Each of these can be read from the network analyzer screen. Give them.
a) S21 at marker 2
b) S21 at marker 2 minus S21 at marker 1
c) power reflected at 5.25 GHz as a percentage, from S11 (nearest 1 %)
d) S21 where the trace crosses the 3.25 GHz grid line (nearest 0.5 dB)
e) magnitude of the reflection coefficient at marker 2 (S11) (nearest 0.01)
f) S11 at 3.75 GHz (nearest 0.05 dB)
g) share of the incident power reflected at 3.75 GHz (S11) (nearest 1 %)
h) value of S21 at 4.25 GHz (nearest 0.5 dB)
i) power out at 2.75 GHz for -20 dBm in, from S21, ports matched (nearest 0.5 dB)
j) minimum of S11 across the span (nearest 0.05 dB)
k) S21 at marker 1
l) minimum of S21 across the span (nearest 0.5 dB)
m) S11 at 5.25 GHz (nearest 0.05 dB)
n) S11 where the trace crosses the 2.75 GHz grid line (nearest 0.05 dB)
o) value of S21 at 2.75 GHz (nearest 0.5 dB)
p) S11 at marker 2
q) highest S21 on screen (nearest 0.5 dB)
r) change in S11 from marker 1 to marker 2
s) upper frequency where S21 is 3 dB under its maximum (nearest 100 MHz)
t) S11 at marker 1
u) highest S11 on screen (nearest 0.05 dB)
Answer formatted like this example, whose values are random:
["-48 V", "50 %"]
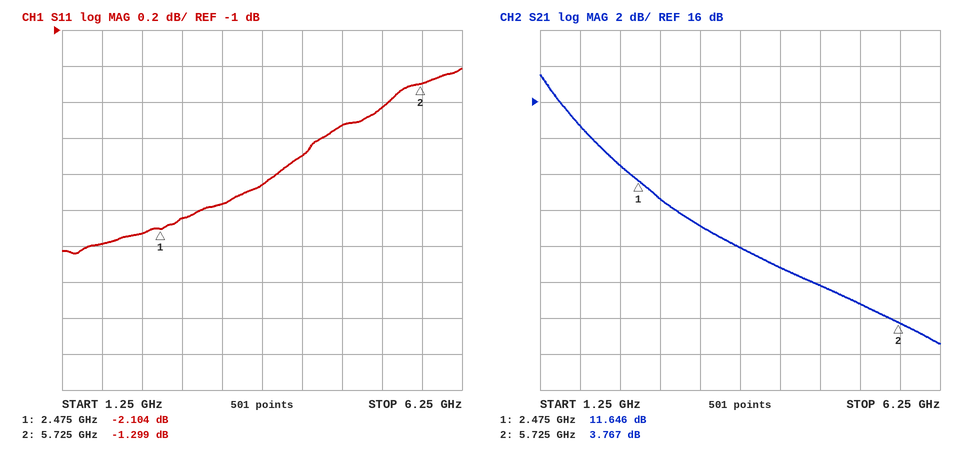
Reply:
["3.767 dB", "-7.879 dB", "72 %", "9.0 dB", "0.86", "-1.85 dB", "65 %", "7.0 dB", "-9.5 dBm", "-2.25 dB", "11.646 dB", "2.5 dB", "-1.45 dB", "-2.05 dB", "10.5 dB", "-1.299 dB", "17.5 dB", "0.805 dB", "1.8 GHz", "-2.104 dB", "-1.20 dB"]
